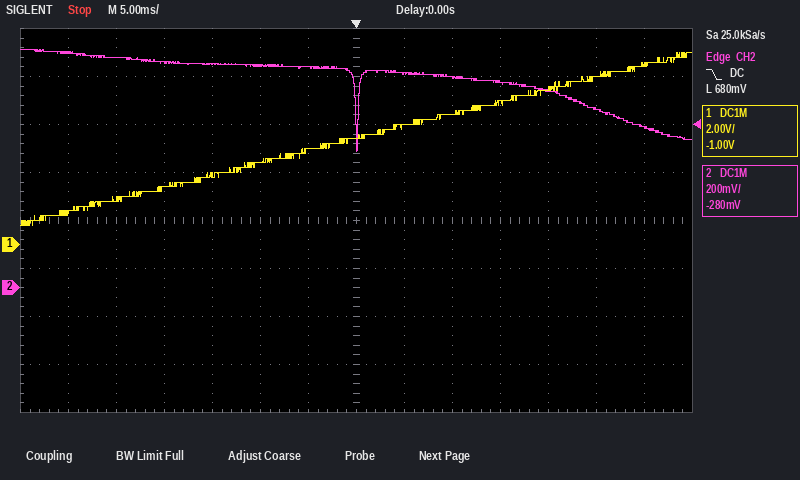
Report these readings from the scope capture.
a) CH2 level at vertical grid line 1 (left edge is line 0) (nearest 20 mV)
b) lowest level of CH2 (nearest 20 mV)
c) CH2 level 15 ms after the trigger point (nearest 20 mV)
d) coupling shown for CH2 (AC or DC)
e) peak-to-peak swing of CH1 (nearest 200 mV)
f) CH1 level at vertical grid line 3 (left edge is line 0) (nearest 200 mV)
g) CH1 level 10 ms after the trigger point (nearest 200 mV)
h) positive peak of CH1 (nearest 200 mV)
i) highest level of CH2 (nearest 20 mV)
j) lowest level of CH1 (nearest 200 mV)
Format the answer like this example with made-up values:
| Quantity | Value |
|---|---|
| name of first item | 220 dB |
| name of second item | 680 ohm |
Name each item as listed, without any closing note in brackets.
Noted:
| Quantity | Value |
|---|---|
| CH2 level at vertical grid line 1 (left edge is line 0) | 980 mV |
| lowest level of CH2 | 560 mV |
| CH2 level 15 ms after the trigger point | 860 mV |
| coupling shown for CH2 | DC |
| peak-to-peak swing of CH1 | 7.2 V |
| CH1 level at vertical grid line 3 (left edge is line 0) | 2.4 V |
| CH1 level 10 ms after the trigger point | 5.4 V |
| positive peak of CH1 | 8.0 V |
| highest level of CH2 | 1.00 V |
| lowest level of CH1 | 800 mV |
